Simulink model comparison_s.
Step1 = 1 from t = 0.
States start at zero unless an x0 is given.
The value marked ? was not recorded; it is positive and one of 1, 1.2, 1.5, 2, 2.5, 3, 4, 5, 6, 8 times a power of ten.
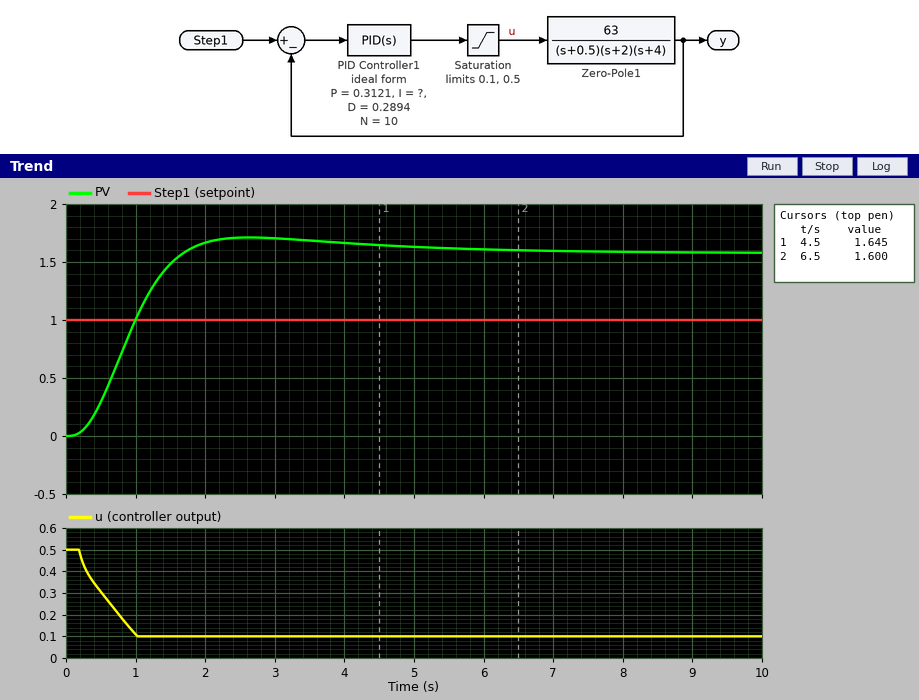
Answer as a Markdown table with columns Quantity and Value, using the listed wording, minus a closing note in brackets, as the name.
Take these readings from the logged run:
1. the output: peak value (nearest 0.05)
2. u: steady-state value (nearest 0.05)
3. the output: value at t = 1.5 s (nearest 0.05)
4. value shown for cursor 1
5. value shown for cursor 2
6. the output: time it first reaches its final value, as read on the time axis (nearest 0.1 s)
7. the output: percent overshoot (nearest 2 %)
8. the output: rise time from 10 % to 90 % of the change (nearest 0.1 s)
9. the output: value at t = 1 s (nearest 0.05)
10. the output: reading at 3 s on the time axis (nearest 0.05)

| Quantity | Value |
|---|---|
| the output: peak value | 1.70 |
| u: steady-state value | 0.10 |
| the output: value at t = 1.5 s | 1.50 |
| value shown for cursor 1 | 1.645 |
| value shown for cursor 2 | 1.600 |
| the output: time it first reaches its final value, as read on the time axis | 1.7 s |
| the output: percent overshoot | 8 % |
| the output: rise time from 10 % to 90 % of the change | 1.0 s |
| the output: value at t = 1 s | 1.00 |
| the output: reading at 3 s on the time axis | 1.70 |
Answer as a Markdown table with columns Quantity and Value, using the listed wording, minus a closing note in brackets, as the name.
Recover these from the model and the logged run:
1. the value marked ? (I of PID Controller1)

| Quantity | Value |
|---|---|
| the value marked ? | 1.2 |
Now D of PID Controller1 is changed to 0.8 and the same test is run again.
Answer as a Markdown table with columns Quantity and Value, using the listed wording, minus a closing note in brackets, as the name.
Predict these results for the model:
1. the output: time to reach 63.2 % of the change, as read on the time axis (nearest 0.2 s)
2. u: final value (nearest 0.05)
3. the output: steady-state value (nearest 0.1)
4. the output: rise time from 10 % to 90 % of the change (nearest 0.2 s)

| Quantity | Value |
|---|---|
| the output: time to reach 63.2 % of the change, as read on the time axis | 1.2 s |
| u: final value | 0.10 |
| the output: steady-state value | 1.6 |
| the output: rise time from 10 % to 90 % of the change | 2.0 s |
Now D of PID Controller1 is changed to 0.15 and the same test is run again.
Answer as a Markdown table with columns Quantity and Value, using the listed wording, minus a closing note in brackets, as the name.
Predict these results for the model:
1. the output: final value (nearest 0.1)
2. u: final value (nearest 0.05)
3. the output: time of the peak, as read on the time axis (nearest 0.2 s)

| Quantity | Value |
|---|---|
| the output: final value | 1.6 |
| u: final value | 0.10 |
| the output: time of the peak, as read on the time axis | 2.4 s |
